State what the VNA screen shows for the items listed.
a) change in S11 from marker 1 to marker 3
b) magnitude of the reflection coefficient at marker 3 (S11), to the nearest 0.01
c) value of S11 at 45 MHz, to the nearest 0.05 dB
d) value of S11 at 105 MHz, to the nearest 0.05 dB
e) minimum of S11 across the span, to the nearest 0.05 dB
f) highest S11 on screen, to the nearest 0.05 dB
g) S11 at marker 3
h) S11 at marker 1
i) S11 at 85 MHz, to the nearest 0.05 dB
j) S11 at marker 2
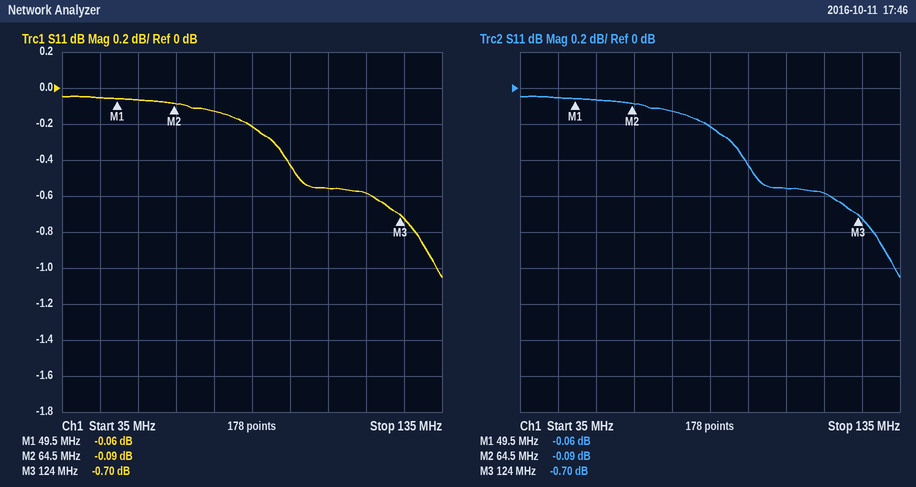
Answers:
-0.64 dB
0.92
-0.05 dB
-0.55 dB
-1.05 dB
-0.05 dB
-0.70 dB
-0.06 dB
-0.20 dB
-0.09 dB
